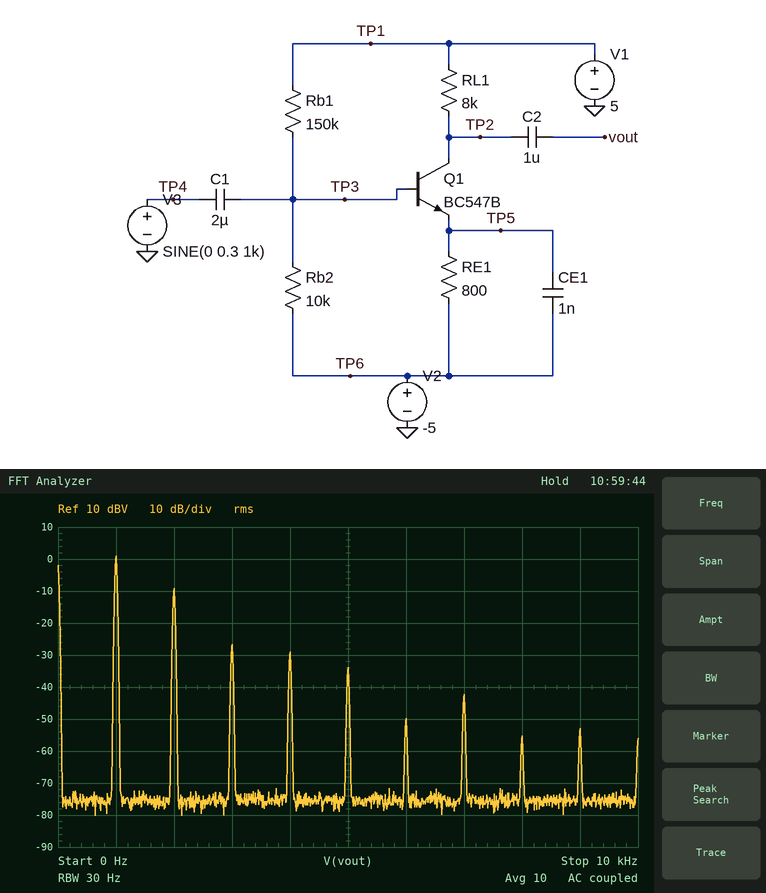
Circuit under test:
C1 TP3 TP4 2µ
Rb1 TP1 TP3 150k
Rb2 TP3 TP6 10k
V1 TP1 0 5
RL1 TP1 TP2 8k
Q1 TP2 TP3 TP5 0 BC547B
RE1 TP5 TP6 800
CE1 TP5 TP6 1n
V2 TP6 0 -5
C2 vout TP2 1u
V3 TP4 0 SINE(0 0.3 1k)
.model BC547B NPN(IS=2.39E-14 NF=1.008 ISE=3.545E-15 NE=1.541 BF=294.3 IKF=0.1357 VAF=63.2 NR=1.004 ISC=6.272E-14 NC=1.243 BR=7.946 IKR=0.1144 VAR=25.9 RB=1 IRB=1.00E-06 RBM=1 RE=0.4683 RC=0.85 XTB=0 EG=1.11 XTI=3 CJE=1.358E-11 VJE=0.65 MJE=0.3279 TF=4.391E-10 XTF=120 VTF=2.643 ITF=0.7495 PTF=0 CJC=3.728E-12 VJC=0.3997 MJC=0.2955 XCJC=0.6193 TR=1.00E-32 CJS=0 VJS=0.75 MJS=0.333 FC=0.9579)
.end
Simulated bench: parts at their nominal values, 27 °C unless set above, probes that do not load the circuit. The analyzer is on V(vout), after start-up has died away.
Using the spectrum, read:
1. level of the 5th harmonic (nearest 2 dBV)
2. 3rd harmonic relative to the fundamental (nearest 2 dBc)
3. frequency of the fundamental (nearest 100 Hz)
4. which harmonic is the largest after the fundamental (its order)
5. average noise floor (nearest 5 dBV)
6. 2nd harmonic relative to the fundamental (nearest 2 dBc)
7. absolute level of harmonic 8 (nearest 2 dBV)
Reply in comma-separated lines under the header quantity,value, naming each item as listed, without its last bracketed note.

quantity,value
level of the 5th harmonic,-34 dBV
3rd harmonic relative to the fundamental,-28 dBc
frequency of the fundamental,1.0 kHz
which harmonic is the largest after the fundamental,2
average noise floor,-75 dBV
2nd harmonic relative to the fundamental,-10 dBc
absolute level of harmonic 8,-56 dBV
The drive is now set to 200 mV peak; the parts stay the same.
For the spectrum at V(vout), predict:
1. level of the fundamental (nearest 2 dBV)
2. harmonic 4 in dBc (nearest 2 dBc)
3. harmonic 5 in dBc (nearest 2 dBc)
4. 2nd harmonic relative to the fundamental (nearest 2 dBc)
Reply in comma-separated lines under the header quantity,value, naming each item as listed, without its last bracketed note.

quantity,value
level of the fundamental,-2 dBV
harmonic 4 in dBc,-40 dBc
harmonic 5 in dBc,-40 dBc
2nd harmonic relative to the fundamental,-12 dBc
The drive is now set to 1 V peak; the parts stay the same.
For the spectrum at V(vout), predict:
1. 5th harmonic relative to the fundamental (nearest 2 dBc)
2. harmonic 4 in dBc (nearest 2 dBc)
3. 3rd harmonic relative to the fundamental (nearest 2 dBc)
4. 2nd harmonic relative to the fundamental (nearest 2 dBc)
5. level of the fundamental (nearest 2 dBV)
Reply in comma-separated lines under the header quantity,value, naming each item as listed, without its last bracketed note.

quantity,value
5th harmonic relative to the fundamental,-42 dBc
harmonic 4 in dBc,-22 dBc
3rd harmonic relative to the fundamental,-44 dBc
2nd harmonic relative to the fundamental,-8 dBc
level of the fundamental,10 dBV
